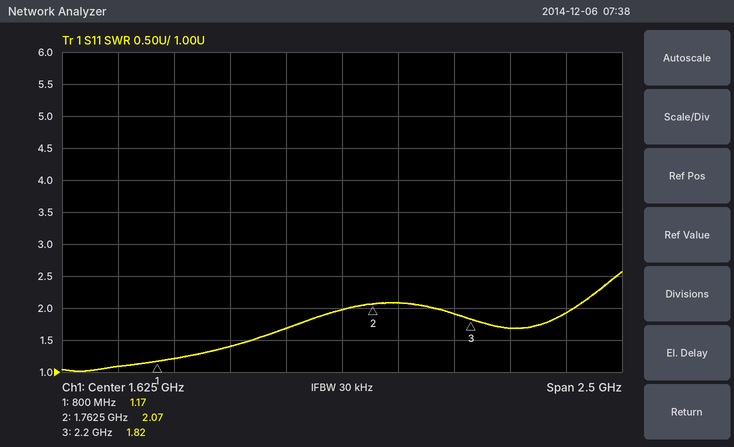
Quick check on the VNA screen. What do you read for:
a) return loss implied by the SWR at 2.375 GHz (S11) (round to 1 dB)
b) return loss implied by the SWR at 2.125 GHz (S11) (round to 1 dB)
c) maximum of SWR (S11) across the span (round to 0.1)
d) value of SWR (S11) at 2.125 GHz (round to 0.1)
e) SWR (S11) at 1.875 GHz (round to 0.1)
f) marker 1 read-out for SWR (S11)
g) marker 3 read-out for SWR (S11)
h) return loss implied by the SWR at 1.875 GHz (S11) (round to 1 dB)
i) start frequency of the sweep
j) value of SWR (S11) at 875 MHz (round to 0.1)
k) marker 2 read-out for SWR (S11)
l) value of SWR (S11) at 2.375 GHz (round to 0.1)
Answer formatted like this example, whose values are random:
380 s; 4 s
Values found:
12 dB; 10 dB; 2.6; 1.9; 2.1; 1.17; 1.82; 9 dB; 375 MHz; 1.2; 2.07; 1.7
